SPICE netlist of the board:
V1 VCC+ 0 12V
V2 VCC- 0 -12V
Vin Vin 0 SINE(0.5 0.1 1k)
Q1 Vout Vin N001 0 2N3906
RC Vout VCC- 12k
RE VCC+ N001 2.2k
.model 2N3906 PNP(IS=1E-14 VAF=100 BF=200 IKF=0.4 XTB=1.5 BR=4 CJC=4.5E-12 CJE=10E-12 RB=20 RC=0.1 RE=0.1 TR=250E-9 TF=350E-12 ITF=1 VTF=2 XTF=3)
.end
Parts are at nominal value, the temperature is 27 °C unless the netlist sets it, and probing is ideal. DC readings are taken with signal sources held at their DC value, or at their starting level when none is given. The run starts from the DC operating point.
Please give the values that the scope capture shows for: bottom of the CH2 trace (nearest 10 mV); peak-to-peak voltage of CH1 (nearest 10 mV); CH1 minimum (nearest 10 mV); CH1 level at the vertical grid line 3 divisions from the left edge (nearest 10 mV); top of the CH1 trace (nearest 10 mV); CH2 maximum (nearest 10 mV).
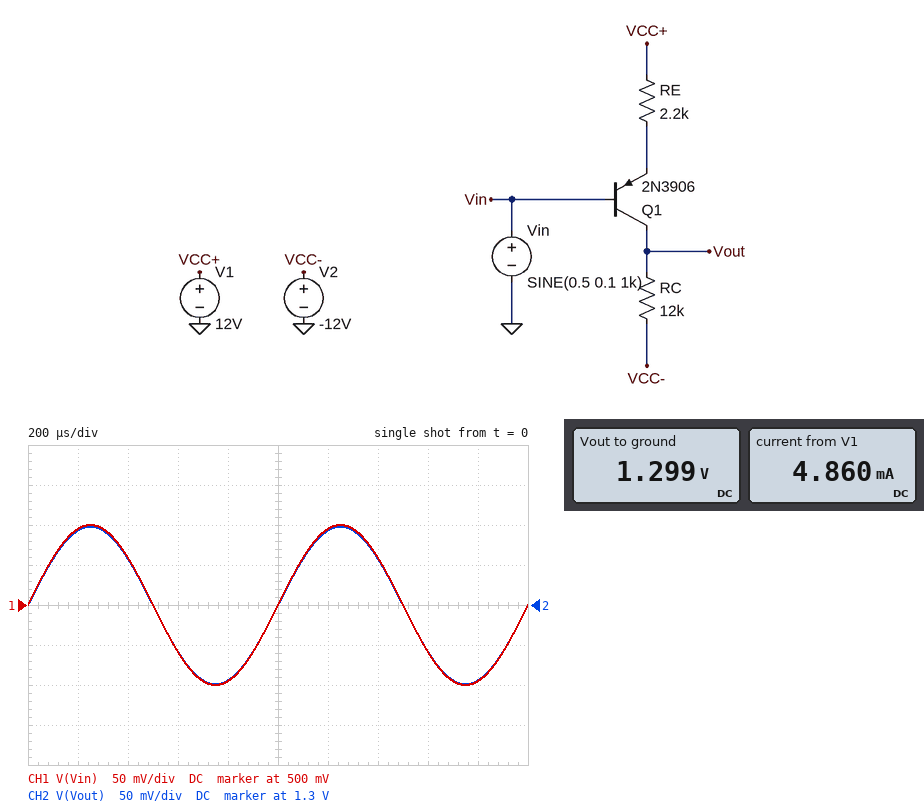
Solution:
1.20 V
200 mV
400 mV
440 mV
600 mV
1.40 V
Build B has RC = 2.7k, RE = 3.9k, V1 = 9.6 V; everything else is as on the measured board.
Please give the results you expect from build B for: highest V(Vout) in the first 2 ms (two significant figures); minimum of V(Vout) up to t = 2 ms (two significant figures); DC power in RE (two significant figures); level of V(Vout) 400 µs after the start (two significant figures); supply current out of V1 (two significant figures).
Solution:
-6.1 V
-6.3 V
18 mW
-6.2 V
2.2 mA
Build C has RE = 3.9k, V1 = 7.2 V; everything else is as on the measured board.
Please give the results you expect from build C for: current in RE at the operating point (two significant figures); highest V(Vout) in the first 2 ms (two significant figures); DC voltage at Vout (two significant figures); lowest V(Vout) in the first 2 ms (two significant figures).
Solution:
1.5 mA
1.3 V
1.2 V
1.1 V
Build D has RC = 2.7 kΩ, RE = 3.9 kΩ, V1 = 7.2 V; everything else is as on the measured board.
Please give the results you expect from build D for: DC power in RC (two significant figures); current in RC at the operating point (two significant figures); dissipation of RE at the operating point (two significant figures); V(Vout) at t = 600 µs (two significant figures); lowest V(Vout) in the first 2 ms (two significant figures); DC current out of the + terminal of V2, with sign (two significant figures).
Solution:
6.4 mW
1.5 mA
9.3 mW
-7.8 V
-7.9 V
-1.5 mA
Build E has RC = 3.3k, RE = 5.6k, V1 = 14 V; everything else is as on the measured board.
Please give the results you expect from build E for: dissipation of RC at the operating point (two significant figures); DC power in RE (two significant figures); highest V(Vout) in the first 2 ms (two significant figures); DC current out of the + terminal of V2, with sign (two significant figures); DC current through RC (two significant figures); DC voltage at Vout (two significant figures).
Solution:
17 mW
29 mW
-4.4 V
-2.3 mA
2.3 mA
-4.5 V
